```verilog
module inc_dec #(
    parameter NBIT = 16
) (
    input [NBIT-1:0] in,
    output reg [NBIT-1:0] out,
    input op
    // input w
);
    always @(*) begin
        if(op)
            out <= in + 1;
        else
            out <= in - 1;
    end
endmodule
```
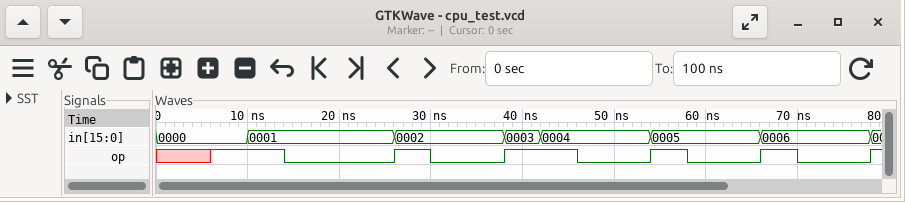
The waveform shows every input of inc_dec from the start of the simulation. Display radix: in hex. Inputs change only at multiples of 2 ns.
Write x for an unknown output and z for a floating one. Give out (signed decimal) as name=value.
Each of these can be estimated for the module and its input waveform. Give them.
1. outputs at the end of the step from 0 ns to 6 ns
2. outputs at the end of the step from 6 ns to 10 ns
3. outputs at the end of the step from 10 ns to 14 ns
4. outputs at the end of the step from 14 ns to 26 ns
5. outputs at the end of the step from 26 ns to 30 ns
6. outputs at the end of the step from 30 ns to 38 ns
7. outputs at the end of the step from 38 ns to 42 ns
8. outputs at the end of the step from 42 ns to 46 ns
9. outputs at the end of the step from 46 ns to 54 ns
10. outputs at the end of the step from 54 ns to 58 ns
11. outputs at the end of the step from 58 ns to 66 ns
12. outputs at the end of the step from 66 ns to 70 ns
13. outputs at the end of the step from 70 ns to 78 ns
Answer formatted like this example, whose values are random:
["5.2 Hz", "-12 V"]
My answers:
["out=-1", "out=1", "out=2", "out=0", "out=3", "out=1", "out=4", "out=5", "out=3", "out=6", "out=4", "out=7", "out=5"]
